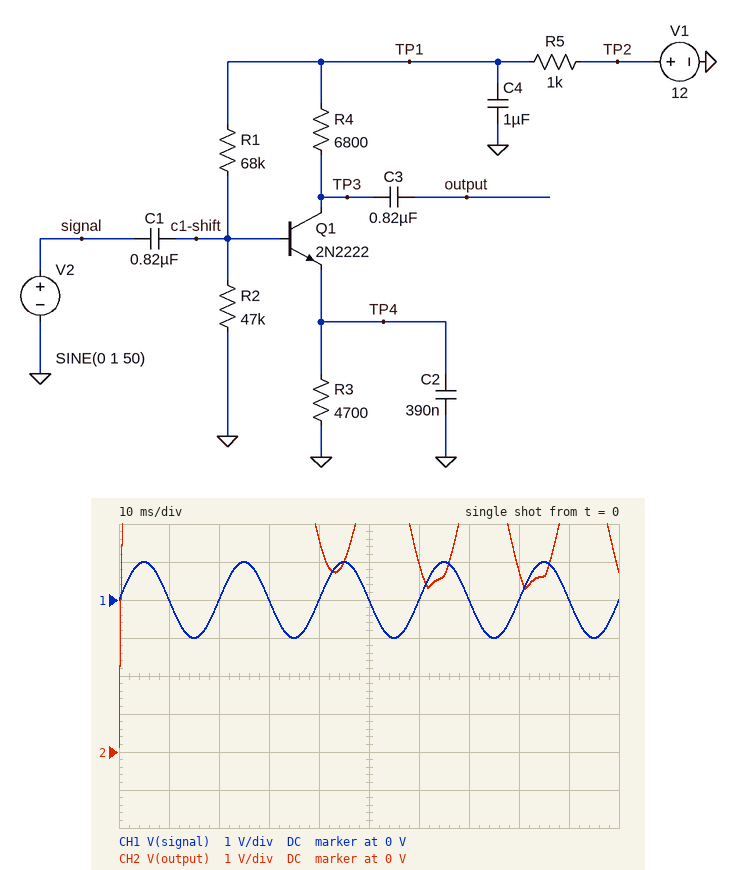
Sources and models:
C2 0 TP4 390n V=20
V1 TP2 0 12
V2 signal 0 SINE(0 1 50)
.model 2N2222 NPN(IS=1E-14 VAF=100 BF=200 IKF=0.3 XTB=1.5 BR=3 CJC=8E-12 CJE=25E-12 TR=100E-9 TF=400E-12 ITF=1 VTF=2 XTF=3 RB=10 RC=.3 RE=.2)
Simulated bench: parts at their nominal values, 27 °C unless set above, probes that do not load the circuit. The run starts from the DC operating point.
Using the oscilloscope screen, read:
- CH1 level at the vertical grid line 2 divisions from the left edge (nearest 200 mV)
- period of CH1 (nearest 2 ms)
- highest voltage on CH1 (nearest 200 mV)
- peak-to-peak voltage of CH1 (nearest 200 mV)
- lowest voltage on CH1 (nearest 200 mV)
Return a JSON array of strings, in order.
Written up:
["0 V", "20 ms", "1.0 V", "2.0 V", "-1.0 V"]
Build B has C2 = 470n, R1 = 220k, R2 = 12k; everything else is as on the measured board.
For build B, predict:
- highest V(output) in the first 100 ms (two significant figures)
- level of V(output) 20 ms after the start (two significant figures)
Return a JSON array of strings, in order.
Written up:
["12 V", "11 V"]
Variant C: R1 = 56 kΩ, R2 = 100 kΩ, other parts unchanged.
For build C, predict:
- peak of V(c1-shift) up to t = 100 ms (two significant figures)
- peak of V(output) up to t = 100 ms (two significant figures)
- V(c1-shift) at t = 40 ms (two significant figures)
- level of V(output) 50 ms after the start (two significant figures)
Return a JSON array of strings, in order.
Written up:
["5.6 V", "10 V", "5.2 V", "5.9 V"]
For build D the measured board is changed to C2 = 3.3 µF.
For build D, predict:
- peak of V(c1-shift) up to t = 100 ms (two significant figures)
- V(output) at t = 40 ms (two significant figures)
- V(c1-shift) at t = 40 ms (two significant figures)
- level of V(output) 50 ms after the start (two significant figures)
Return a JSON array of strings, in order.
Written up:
["4.4 V", "2.8 V", "3.4 V", "12 V"]
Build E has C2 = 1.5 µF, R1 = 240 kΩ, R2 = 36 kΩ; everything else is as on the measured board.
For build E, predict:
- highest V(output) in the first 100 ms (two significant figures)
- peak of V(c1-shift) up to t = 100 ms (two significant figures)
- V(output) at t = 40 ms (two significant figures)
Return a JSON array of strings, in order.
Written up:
["12 V", "2.4 V", "7.4 V"]
